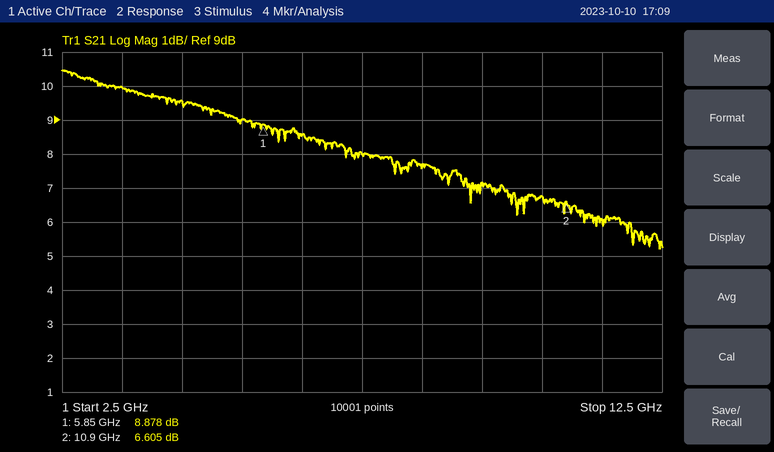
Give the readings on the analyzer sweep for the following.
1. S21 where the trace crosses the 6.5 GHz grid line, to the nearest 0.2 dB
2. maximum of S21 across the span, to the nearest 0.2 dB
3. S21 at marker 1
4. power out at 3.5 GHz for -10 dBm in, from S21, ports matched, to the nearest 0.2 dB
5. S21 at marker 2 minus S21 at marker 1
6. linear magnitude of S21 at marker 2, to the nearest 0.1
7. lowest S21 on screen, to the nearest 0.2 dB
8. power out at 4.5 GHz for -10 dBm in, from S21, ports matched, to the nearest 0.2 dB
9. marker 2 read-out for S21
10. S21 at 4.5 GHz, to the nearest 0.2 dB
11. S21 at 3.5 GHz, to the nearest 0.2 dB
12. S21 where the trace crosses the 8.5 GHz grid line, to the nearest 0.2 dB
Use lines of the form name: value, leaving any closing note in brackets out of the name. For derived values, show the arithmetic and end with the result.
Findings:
S21 where the trace crosses the 6.5 GHz grid line, to the nearest 0.2 dB: 8.6 dB
maximum of S21 across the span, to the nearest 0.2 dB: 10.4 dB
S21 at marker 1: 8.878 dB
power out at 3.5 GHz for -10 dBm in, from S21, ports matched, to the nearest 0.2 dB: -10 dBm + (10.0 dB) = 0.0 dBm
S21 at marker 2 minus S21 at marker 1: 6.605 − (8.878) = -2.273 dB
linear magnitude of S21 at marker 2, to the nearest 0.1: 10^(6.605/20) ≈ 2.1
lowest S21 on screen, to the nearest 0.2 dB: 5.2 dB
power out at 4.5 GHz for -10 dBm in, from S21, ports matched, to the nearest 0.2 dB: -10 dBm + (9.6 dB) = -0.4 dBm
marker 2 read-out for S21: 6.605 dB
S21 at 4.5 GHz, to the nearest 0.2 dB: 9.6 dB
S21 at 3.5 GHz, to the nearest 0.2 dB: 10.0 dB
S21 where the trace crosses the 8.5 GHz grid line, to the nearest 0.2 dB: 7.6 dB
